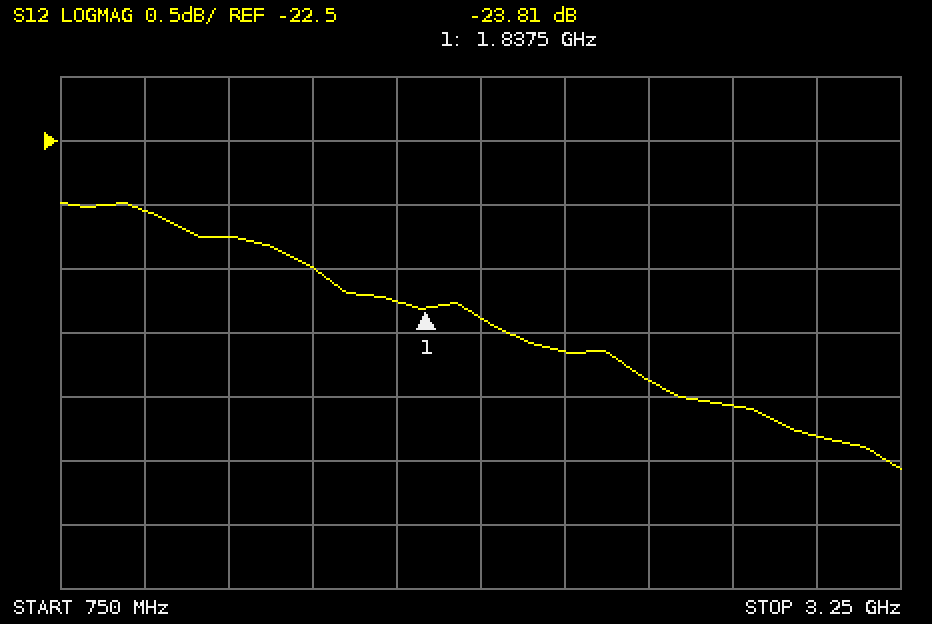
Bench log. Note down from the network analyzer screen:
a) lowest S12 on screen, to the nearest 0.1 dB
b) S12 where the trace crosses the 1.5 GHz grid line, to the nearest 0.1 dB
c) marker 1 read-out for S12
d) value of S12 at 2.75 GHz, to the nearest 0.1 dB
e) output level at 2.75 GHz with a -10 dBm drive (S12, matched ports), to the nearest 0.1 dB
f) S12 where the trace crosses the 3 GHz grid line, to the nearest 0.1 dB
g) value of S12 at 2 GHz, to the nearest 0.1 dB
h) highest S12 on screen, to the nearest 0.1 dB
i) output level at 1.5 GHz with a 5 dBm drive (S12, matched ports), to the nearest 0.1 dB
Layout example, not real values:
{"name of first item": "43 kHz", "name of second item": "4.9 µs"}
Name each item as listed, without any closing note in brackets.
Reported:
{"lowest S12 on screen, to the nearest 0.1 dB": "-25.1 dB", "S12 where the trace crosses the 1.5 GHz grid line, to the nearest 0.1 dB": "-23.5 dB", "marker 1 read-out for S12": "-23.81 dB", "value of S12 at 2.75 GHz, to the nearest 0.1 dB": "-24.6 dB", "output level at 2.75 GHz with a -10 dBm drive (S12, matched ports), to the nearest 0.1 dB": "-34.6 dBm", "S12 where the trace crosses the 3 GHz grid line, to the nearest 0.1 dB": "-24.8 dB", "value of S12 at 2 GHz, to the nearest 0.1 dB": "-23.9 dB", "highest S12 on screen, to the nearest 0.1 dB": "-23.0 dB", "output level at 1.5 GHz with a 5 dBm drive (S12, matched ports), to the nearest 0.1 dB": "-18.5 dBm"}
